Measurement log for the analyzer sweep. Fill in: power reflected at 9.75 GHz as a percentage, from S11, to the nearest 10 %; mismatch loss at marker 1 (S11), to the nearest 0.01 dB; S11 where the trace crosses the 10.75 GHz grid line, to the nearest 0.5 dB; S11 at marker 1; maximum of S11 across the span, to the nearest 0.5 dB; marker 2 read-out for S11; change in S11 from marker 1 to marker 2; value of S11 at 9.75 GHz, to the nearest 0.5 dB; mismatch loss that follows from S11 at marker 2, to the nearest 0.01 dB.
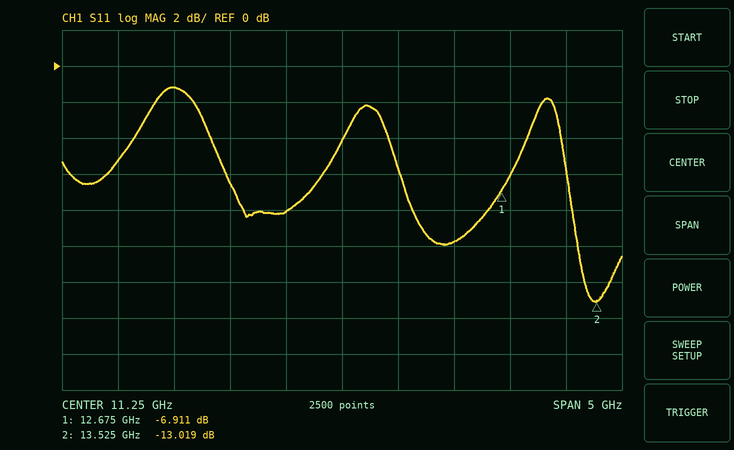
80 %
0.99 dB
-8.0 dB
-6.911 dB
-1.0 dB
-13.019 dB
-6.108 dB
-1.0 dB
0.22 dB
